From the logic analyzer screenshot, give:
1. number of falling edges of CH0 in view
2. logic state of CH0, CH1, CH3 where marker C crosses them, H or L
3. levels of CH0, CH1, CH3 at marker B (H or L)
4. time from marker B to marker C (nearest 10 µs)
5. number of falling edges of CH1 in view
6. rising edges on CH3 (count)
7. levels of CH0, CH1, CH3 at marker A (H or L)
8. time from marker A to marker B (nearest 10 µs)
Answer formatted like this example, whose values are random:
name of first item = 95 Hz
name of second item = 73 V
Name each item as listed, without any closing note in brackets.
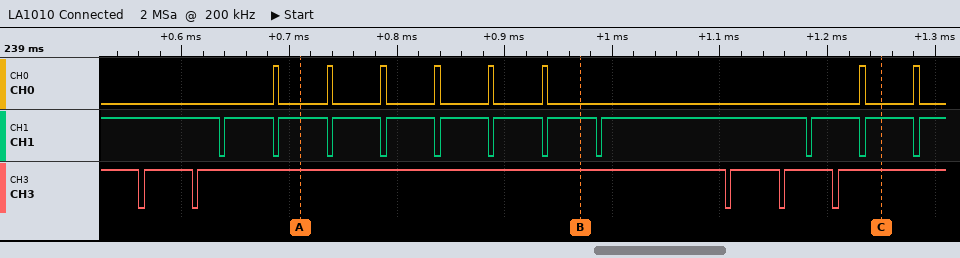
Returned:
number of falling edges of CH0 in view = 8
logic state of CH0, CH1, CH3 where marker C crosses them, H or L = CH0=L, CH1=H, CH3=H
levels of CH0, CH1, CH3 at marker B = CH0=L, CH1=H, CH3=H
time from marker B to marker C = 280 µs
number of falling edges of CH1 in view = 11
rising edges on CH3 = 5
levels of CH0, CH1, CH3 at marker A = CH0=L, CH1=H, CH3=H
time from marker A to marker B = 260 µs
